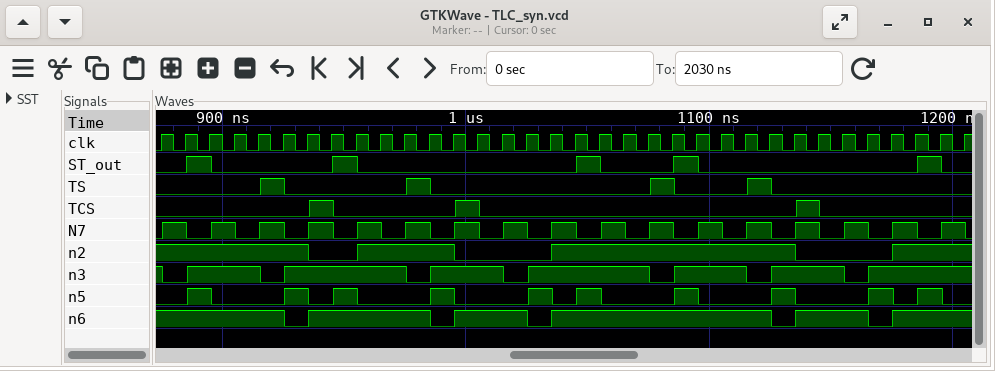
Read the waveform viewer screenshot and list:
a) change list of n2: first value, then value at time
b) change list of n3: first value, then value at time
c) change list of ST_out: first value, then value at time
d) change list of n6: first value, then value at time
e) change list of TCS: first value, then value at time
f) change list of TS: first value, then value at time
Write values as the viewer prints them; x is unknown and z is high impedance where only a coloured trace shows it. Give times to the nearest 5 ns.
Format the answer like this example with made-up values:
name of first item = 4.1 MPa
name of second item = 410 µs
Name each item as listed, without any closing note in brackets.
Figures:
change list of n2: first value, then value at time = 1, 0 at 935 ns, 1 at 955 ns, 0 at 995 ns, 1 at 1035 ns, 0 at 1135 ns, 1 at 1175 ns
change list of n3: first value, then value at time = 1, 0 at 875 ns, 1 at 885 ns, 0 at 915 ns, 1 at 925 ns, 0 at 975 ns, 1 at 985 ns, 0 at 1015 ns, 1 at 1025 ns, 0 at 1075 ns, 1 at 1085 ns, 0 at 1115 ns, 1 at 1125 ns, 0 at 1155 ns, 1 at 1165 ns
change list of ST_out: first value, then value at time = 0, 1 at 885 ns, 0 at 895 ns, 1 at 945 ns, 0 at 955 ns, 1 at 1045 ns, 0 at 1055 ns, 1 at 1085 ns, 0 at 1095 ns, 1 at 1185 ns, 0 at 1195 ns
change list of n6: first value, then value at time = 1, 0 at 925 ns, 1 at 935 ns, 0 at 985 ns, 1 at 995 ns, 0 at 1025 ns, 1 at 1035 ns, 0 at 1125 ns, 1 at 1135 ns, 0 at 1165 ns, 1 at 1175 ns
change list of TCS: first value, then value at time = 0, 1 at 935 ns, 0 at 945 ns, 1 at 995 ns, 0 at 1005 ns, 1 at 1135 ns, 0 at 1145 ns
change list of TS: first value, then value at time = 0, 1 at 915 ns, 0 at 925 ns, 1 at 975 ns, 0 at 985 ns, 1 at 1075 ns, 0 at 1085 ns, 1 at 1115 ns, 0 at 1125 ns
